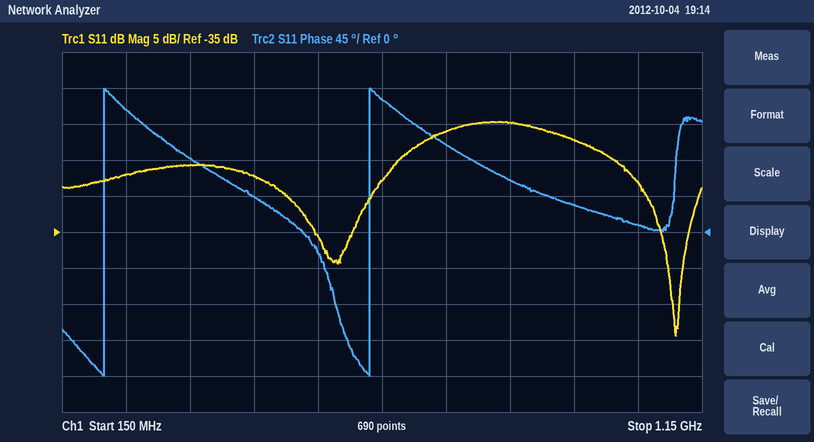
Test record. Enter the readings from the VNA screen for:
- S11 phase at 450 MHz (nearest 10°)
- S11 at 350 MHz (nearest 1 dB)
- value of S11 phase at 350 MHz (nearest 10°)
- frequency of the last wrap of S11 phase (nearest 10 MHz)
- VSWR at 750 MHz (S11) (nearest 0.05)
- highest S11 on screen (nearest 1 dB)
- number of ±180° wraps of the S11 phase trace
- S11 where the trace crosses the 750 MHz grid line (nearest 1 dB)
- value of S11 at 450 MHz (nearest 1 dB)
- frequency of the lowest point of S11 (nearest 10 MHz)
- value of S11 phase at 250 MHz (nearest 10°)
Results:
40°
-26 dB
90°
630 MHz
1.20
-20 dB
2
-21 dB
-27 dB
1.11 GHz
150°
